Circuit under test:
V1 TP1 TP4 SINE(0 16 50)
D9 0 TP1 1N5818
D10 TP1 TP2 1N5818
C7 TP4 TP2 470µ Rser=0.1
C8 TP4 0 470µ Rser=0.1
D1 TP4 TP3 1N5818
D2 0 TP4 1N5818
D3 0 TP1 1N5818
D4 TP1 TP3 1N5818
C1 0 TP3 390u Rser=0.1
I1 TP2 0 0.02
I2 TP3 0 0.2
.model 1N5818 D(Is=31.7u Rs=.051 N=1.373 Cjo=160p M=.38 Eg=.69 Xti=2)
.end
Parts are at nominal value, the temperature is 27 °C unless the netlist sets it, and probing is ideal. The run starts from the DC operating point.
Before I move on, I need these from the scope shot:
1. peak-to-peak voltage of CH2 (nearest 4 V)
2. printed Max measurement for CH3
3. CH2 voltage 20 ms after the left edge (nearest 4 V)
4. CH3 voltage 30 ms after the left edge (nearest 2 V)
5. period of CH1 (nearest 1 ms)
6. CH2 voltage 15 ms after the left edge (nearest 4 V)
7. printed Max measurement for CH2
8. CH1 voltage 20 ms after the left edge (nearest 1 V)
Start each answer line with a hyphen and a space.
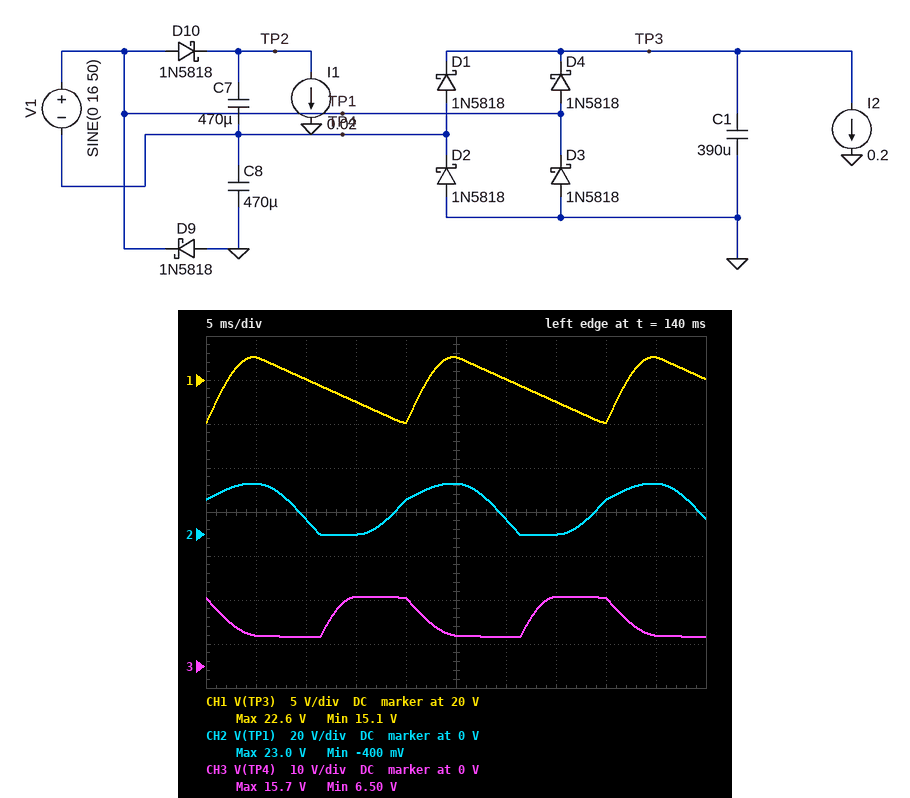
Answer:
- 24 V
- 15.7 V
- 16 V
- 6 V
- 20 ms
- 0 V
- 23.0 V
- 15 V
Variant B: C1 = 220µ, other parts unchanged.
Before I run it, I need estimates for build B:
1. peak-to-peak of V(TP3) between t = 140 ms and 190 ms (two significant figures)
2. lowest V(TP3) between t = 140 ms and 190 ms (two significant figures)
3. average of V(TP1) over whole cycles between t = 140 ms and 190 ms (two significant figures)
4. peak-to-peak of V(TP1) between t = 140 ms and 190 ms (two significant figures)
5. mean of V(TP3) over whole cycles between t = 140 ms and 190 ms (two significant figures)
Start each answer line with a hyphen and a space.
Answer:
- 9.3 V
- 14 V
- 11 V
- 24 V
- 18 V
